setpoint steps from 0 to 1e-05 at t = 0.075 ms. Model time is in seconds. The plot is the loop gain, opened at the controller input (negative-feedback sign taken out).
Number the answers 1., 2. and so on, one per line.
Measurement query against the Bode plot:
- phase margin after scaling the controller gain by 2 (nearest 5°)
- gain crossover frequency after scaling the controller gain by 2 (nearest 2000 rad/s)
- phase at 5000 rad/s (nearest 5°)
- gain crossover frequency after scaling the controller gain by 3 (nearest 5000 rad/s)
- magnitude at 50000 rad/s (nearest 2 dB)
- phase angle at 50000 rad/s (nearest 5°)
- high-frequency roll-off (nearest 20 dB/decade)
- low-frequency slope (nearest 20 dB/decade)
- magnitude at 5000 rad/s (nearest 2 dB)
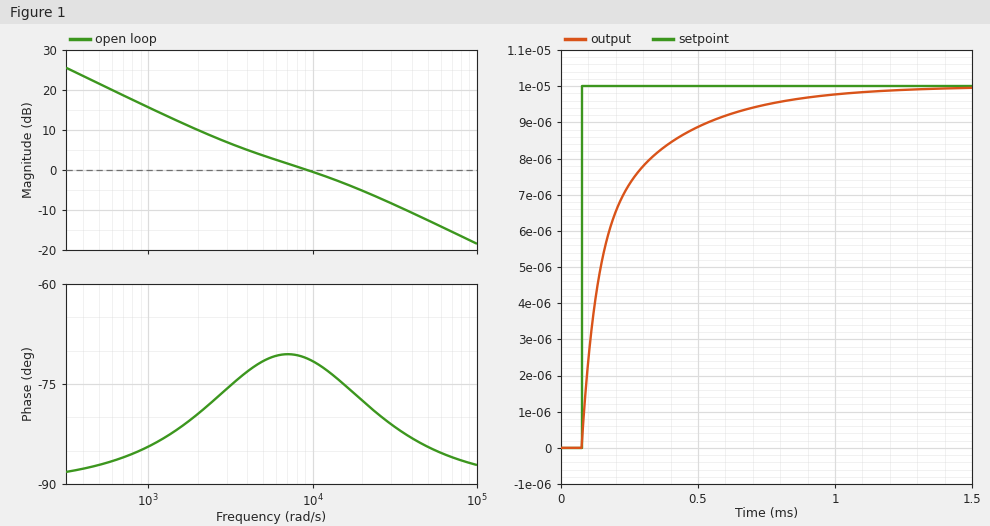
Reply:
1. 100°
2. 22000 rad/s
3. -70°
4. 35000 rad/s
5. -12 dB
6. -85°
7. -20 dB/decade
8. -20 dB/decade
9. 4 dB
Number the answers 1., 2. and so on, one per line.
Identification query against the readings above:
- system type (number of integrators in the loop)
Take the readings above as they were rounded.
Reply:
1. 1
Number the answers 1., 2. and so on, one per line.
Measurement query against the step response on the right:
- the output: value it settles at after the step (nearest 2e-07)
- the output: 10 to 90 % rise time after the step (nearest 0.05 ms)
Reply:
1. 0.0000100
2. 0.45 ms
